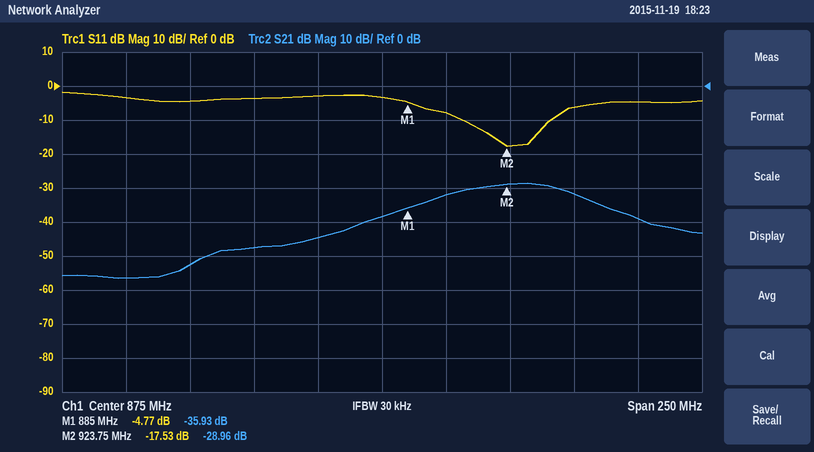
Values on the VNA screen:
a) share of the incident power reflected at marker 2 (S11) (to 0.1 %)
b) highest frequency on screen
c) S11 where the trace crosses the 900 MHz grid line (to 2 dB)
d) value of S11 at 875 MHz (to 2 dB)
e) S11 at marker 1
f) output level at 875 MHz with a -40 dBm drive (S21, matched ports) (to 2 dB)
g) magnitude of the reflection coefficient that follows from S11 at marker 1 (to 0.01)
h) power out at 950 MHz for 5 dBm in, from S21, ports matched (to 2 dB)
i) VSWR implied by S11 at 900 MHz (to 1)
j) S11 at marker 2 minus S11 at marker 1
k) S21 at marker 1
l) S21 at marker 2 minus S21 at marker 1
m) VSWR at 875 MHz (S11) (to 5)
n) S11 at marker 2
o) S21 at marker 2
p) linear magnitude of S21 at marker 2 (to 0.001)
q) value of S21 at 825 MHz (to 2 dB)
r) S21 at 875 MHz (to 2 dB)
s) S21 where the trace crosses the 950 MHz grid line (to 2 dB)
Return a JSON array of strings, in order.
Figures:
["1.8 %", "1 GHz", "-8 dB", "-4 dB", "-4.77 dB", "-78 dBm", "0.58", "-26 dBm", "2", "-12.76 dB", "-35.93 dB", "6.97 dB", "5", "-17.53 dB", "-28.96 dB", "0.036", "-48 dB", "-38 dB", "-32 dB"]
